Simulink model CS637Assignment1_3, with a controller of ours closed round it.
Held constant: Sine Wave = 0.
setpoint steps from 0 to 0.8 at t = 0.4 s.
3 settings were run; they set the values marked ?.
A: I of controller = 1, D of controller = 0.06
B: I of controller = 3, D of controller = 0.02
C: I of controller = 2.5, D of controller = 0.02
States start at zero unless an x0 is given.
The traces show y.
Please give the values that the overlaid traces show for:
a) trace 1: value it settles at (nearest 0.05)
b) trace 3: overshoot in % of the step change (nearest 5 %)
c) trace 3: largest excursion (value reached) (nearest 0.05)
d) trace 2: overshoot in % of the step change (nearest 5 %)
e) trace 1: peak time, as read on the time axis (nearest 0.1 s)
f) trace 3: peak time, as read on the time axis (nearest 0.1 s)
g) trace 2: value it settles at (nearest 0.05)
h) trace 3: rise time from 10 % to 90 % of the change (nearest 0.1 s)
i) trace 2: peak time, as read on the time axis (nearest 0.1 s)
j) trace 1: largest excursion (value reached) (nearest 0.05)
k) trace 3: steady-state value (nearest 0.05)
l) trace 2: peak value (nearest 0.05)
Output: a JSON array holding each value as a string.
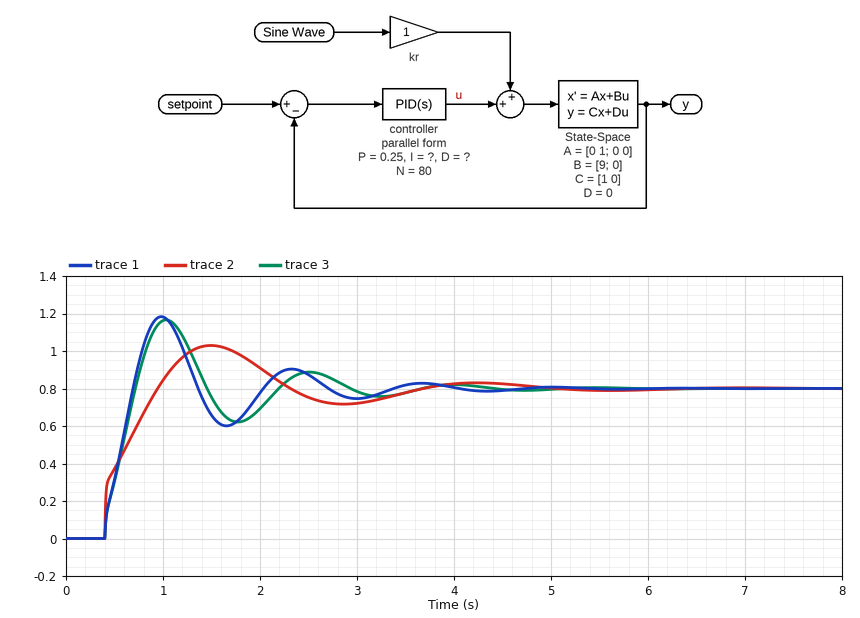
["0.80", "45 %", "1.15", "30 %", "1.0 s", "1.0 s", "0.80", "0.3 s", "1.5 s", "1.20", "0.80", "1.05"]
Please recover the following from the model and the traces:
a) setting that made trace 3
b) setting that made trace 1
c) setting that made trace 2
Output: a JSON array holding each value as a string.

["C", "B", "A"]
